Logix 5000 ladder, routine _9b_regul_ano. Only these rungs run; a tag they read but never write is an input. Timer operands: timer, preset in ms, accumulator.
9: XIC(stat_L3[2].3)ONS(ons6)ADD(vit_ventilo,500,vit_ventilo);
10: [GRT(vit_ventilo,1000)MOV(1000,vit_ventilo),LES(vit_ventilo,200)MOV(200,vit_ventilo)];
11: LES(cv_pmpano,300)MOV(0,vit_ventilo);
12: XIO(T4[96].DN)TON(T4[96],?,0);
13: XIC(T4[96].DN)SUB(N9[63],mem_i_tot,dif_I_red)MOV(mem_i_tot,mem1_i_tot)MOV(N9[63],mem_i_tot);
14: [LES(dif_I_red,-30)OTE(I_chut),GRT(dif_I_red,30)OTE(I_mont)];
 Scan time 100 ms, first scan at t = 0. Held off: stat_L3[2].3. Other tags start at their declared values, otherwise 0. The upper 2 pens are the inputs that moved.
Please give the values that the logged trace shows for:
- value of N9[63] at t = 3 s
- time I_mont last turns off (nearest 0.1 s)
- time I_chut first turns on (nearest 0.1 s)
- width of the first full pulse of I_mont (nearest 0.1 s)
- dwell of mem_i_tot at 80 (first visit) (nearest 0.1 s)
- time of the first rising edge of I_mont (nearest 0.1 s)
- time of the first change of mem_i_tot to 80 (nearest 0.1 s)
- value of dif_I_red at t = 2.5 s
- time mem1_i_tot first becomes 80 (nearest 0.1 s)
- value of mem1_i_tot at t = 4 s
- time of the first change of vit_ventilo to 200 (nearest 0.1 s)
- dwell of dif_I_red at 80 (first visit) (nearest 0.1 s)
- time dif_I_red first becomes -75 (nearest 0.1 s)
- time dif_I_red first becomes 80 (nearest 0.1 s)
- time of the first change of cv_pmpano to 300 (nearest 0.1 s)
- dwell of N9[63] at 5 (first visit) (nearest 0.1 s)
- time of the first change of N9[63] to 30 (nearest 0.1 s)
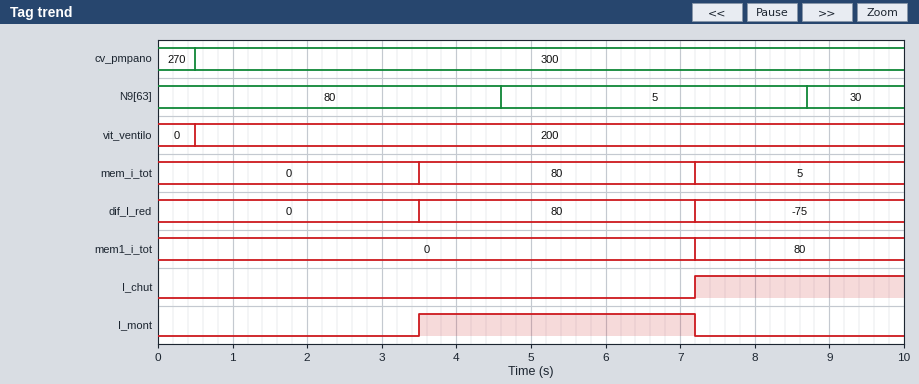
80
7.2 s
7.2 s
3.7 s
3.7 s
3.5 s
3.5 s
0
7.2 s
0
0.5 s
3.7 s
7.2 s
3.5 s
0.5 s
4.1 s
8.7 s
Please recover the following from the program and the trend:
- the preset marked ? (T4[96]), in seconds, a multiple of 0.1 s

3.5 s
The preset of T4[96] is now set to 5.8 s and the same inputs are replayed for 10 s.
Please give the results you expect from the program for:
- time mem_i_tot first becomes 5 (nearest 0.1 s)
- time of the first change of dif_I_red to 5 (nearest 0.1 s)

5.8 s
5.8 s
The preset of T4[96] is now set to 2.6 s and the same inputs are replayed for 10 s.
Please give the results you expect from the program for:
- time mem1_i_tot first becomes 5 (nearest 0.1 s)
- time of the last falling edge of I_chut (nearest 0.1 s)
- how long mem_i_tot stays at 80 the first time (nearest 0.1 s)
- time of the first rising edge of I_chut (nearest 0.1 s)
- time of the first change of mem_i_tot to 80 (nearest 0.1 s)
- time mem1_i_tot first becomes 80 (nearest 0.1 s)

8.2 s
8.2 s
2.8 s
5.4 s
2.6 s
5.4 s
